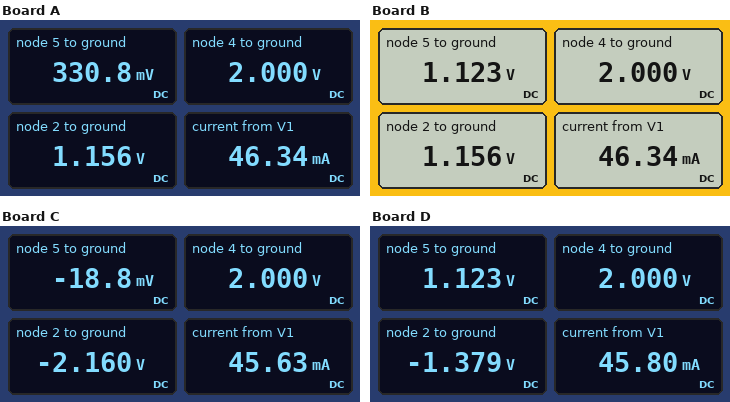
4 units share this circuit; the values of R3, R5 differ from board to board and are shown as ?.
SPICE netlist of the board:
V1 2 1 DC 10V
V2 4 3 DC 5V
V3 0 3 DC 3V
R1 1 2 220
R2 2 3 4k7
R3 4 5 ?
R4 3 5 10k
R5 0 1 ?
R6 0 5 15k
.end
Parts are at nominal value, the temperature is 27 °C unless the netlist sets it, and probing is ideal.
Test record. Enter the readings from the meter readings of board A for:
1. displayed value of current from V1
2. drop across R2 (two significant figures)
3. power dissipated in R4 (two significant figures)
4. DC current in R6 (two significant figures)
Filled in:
46.34 mA
4.2 V
1.1 mW
22 µA
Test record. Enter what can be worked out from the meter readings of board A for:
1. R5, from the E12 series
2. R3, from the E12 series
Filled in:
10 kΩ
4.7 kΩ
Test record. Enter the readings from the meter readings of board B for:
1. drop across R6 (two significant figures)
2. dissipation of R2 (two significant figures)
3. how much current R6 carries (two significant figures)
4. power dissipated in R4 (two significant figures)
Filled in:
1.1 V
3.7 mW
75 µA
1.7 mW
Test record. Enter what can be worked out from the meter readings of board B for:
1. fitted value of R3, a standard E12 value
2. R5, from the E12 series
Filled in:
1.8 kΩ
10 kΩ
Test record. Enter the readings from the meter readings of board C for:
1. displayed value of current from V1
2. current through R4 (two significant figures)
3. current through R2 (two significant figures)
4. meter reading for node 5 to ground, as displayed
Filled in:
45.63 mA
300 µA
180 µA
-18.8 mV
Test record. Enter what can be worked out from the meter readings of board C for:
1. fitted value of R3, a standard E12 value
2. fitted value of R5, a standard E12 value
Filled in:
6.8 kΩ
68 kΩ
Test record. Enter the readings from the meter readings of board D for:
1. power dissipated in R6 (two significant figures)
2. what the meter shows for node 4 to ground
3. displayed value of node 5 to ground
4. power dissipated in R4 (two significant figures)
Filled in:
84 µW
2.000 V
1.123 V
1.7 mW
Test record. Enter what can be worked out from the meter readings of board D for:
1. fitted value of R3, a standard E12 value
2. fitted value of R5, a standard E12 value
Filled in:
1.8 kΩ
33 kΩ
